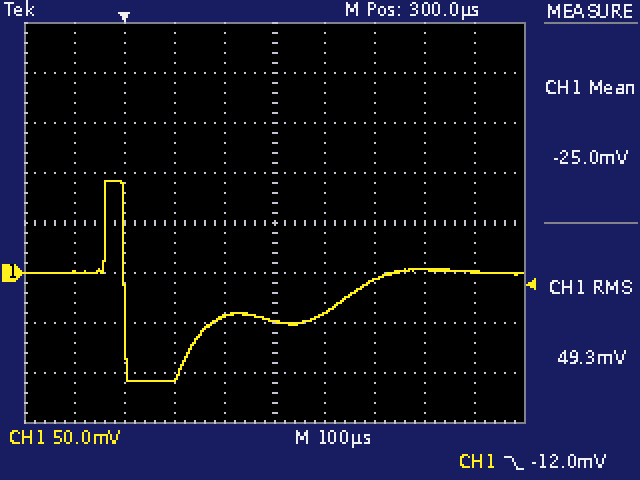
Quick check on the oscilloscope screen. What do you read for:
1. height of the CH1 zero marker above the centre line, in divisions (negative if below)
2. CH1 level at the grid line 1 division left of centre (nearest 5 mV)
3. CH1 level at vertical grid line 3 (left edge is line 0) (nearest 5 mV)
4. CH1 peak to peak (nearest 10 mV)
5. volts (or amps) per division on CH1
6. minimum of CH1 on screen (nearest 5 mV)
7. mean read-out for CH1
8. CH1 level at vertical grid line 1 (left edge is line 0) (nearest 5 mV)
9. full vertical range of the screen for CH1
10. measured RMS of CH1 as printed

-1.0 div
-45 mV
-105 mV
200 mV
50 mV
-110 mV
-25.0 mV
0 mV
400 mV
49.3 mV
